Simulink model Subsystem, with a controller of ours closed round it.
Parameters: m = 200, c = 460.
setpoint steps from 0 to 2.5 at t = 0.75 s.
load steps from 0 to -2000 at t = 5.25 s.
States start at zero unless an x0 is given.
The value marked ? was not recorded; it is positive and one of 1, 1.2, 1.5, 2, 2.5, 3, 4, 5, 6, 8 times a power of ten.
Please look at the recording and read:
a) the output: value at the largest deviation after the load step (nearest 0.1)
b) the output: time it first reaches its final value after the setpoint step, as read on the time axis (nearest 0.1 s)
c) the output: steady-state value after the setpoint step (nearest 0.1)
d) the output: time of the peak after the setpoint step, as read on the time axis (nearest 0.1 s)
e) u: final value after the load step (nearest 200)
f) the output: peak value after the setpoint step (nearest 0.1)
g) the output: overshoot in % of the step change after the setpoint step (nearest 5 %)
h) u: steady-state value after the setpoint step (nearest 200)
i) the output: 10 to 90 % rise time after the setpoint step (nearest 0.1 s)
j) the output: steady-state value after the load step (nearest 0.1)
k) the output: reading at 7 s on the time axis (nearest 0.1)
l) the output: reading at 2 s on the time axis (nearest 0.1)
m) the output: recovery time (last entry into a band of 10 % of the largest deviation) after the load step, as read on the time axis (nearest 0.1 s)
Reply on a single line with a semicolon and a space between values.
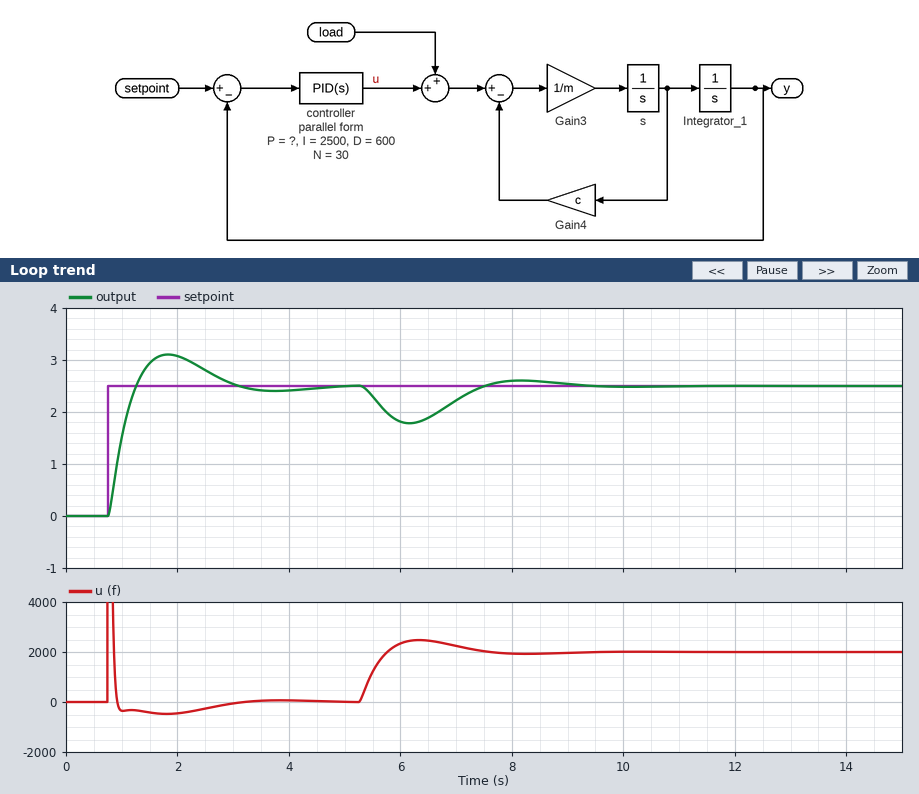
1.8; 1.3 s; 2.5; 1.8 s; 2000; 3.1; 25 %; 0; 0.4 s; 2.5; 2.2; 3.1; 8.7 s
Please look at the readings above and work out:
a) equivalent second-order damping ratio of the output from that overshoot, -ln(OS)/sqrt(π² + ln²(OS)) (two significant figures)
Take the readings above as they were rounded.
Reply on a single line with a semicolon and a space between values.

0.40
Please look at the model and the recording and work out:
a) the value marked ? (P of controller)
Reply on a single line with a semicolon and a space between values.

2000
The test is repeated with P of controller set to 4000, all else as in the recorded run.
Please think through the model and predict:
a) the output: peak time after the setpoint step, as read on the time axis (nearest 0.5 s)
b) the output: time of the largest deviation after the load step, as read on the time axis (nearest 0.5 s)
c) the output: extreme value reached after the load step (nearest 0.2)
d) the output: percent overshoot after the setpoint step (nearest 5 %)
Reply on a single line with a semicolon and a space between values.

1.5 s; 6.0 s; 2.0; 25 %
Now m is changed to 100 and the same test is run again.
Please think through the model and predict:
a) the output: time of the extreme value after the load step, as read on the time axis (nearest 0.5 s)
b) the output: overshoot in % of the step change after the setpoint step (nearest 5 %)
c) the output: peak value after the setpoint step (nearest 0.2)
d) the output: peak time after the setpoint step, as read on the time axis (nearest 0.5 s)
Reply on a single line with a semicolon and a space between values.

6.0 s; 15 %; 2.8; 2.0 s
